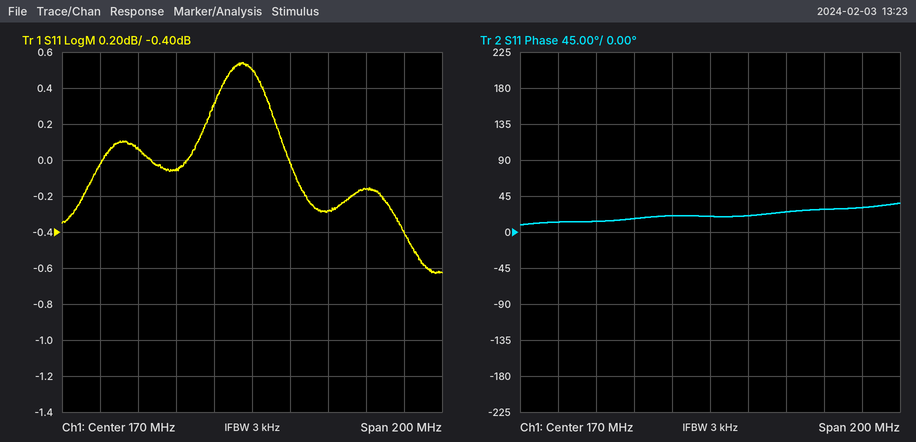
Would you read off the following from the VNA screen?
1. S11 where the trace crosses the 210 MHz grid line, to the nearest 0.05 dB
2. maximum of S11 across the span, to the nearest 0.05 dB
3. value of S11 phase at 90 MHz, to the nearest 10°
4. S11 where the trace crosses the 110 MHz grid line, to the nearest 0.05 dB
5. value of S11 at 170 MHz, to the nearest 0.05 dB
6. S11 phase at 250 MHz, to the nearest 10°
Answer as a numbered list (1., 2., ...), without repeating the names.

1. -0.30 dB
2. 0.55 dB
3. 10°
4. 0.05 dB
5. 0.50 dB
6. 30°
